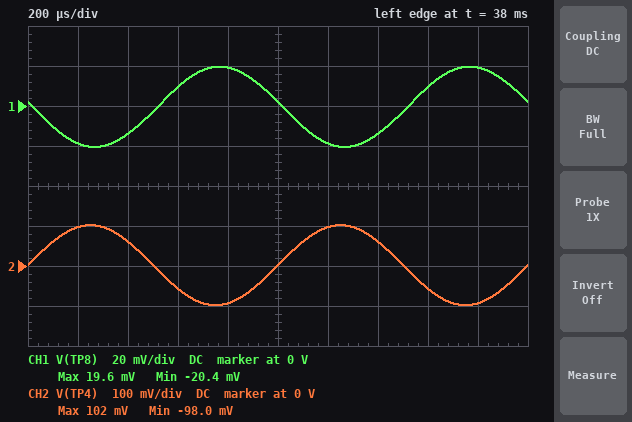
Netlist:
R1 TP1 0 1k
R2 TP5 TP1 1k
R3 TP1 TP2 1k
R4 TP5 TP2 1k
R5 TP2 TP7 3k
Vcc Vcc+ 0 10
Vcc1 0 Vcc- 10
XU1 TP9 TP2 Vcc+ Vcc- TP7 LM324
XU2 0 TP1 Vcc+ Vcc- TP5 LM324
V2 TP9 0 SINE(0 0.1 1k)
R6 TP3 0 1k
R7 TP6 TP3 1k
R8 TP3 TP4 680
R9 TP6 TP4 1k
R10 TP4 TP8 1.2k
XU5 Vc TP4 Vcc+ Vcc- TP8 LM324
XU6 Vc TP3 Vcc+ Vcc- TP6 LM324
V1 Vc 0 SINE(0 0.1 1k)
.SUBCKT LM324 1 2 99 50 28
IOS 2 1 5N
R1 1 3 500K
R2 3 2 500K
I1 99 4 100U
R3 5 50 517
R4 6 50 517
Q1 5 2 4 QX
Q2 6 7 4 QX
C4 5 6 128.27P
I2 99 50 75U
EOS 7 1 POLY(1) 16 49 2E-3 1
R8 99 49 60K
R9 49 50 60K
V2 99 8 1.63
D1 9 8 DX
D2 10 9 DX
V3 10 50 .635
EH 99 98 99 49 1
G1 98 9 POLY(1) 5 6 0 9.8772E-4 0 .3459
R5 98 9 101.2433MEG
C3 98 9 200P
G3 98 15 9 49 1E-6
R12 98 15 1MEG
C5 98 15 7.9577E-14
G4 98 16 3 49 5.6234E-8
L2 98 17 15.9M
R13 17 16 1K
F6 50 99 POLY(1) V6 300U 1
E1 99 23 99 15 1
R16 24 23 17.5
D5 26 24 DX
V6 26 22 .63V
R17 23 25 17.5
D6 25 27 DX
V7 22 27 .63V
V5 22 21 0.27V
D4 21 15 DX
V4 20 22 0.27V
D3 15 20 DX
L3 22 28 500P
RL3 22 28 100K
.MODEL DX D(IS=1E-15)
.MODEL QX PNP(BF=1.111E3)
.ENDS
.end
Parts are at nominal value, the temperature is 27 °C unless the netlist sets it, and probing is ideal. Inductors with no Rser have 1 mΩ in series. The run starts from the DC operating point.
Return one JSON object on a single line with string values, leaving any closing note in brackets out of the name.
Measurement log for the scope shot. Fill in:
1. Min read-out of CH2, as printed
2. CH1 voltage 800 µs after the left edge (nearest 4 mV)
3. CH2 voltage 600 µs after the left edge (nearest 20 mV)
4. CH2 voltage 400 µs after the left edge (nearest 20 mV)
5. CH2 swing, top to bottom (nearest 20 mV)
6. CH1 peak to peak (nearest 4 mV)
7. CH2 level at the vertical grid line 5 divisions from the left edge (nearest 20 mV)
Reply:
{"Min read-out of CH2, as printed": "-98.0 mV", "CH1 voltage 800 µs after the left edge": "20 mV", "CH2 voltage 600 µs after the left edge": "-60 mV", "CH2 voltage 400 µs after the left edge": "60 mV", "CH2 swing, top to bottom": "200 mV", "CH1 peak to peak": "40 mV", "CH2 level at the vertical grid line 5 divisions from the left edge": "0 V"}
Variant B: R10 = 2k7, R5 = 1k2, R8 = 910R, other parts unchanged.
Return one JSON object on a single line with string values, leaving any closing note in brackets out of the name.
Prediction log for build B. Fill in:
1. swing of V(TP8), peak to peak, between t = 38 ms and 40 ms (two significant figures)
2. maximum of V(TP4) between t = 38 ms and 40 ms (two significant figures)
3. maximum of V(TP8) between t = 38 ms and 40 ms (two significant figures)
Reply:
{"swing of V(TP8), peak to peak, between t = 38 ms and 40 ms": "340 mV", "maximum of V(TP4) between t = 38 ms and 40 ms": "100 mV", "maximum of V(TP8) between t = 38 ms and 40 ms": "170 mV"}
